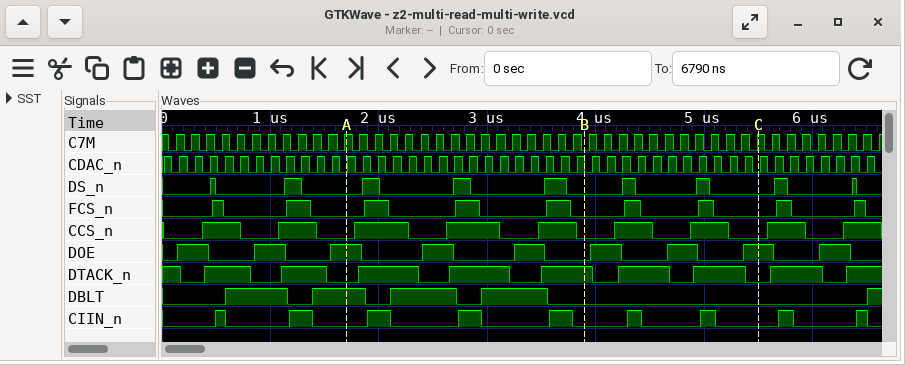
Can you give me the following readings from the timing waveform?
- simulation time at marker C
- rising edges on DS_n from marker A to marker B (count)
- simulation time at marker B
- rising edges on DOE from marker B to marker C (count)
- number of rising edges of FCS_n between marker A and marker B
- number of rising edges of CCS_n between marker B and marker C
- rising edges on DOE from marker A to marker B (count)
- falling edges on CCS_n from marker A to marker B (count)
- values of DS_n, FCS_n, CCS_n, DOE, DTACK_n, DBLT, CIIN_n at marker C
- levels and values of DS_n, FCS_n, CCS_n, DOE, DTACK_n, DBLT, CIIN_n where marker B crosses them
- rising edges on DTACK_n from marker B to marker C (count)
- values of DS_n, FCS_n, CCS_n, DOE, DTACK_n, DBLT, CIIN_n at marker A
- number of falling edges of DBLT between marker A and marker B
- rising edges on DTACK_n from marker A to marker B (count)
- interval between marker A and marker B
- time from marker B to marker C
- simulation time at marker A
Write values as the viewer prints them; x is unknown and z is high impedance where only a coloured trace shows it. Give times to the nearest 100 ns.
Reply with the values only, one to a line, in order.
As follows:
5500 ns
3
3900 ns
3
3
2
2
3
DS_n=0, FCS_n=0, CCS_n=0, DOE=1, DTACK_n=0, DBLT=0, CIIN_n=0
DS_n=0, FCS_n=0, CCS_n=0, DOE=0, DTACK_n=1, DBLT=0, CIIN_n=0
2
DS_n=0, FCS_n=0, CCS_n=0, DOE=1, DTACK_n=0, DBLT=1, CIIN_n=0
3
3
2200 ns
1600 ns
1700 ns
